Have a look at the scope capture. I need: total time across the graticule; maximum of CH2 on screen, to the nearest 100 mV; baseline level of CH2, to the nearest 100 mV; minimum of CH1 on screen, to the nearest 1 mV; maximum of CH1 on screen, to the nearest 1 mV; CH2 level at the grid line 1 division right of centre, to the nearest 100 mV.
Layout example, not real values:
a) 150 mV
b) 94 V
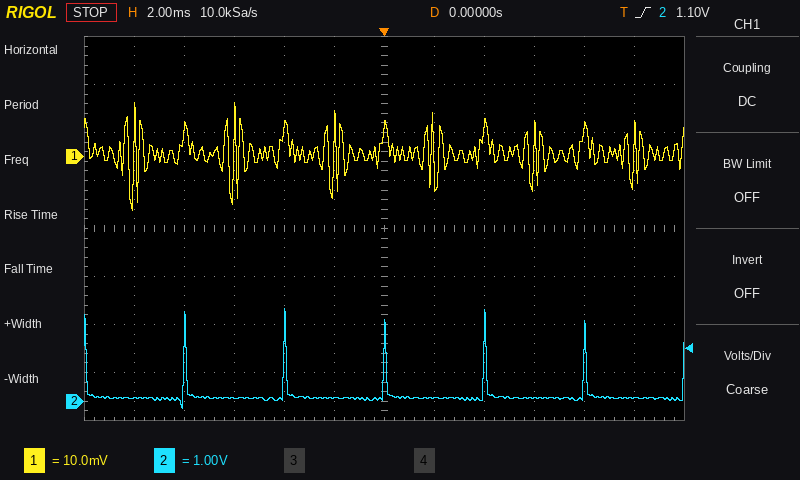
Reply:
a) 24 ms
b) 1.9 V
c) 100 mV
d) -11 mV
e) 11 mV
f) 100 mV
